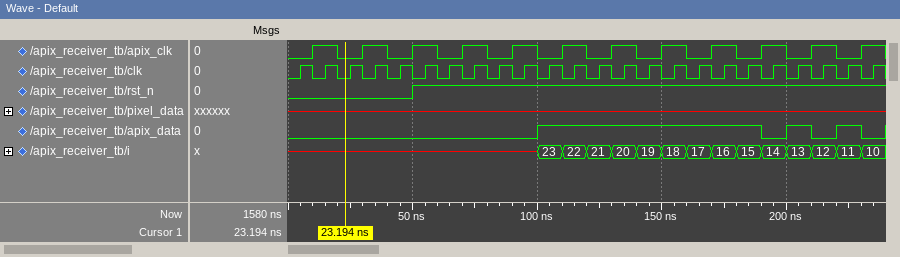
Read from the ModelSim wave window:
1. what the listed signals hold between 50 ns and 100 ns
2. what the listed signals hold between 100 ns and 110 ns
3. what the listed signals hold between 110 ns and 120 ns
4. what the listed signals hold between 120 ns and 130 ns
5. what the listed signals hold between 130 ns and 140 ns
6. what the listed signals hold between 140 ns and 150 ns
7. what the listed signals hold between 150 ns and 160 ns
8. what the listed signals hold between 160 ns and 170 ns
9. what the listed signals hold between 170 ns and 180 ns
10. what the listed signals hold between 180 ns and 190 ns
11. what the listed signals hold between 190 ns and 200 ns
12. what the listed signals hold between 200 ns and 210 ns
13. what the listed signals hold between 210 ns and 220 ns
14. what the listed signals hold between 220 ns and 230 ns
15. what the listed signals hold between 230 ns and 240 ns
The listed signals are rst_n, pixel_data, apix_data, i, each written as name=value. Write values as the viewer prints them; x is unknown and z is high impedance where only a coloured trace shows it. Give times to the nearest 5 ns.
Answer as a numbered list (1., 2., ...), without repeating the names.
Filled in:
1. rst_n=1, pixel_data=x, apix_data=0, i=x
2. rst_n=1, pixel_data=x, apix_data=1, i=23
3. rst_n=1, pixel_data=x, apix_data=1, i=22
4. rst_n=1, pixel_data=x, apix_data=1, i=21
5. rst_n=1, pixel_data=x, apix_data=1, i=20
6. rst_n=1, pixel_data=x, apix_data=1, i=19
7. rst_n=1, pixel_data=x, apix_data=1, i=18
8. rst_n=1, pixel_data=x, apix_data=1, i=17
9. rst_n=1, pixel_data=x, apix_data=1, i=16
10. rst_n=1, pixel_data=x, apix_data=1, i=15
11. rst_n=1, pixel_data=x, apix_data=0, i=14
12. rst_n=1, pixel_data=x, apix_data=1, i=13
13. rst_n=1, pixel_data=x, apix_data=0, i=12
14. rst_n=1, pixel_data=x, apix_data=1, i=11
15. rst_n=1, pixel_data=x, apix_data=0, i=10
